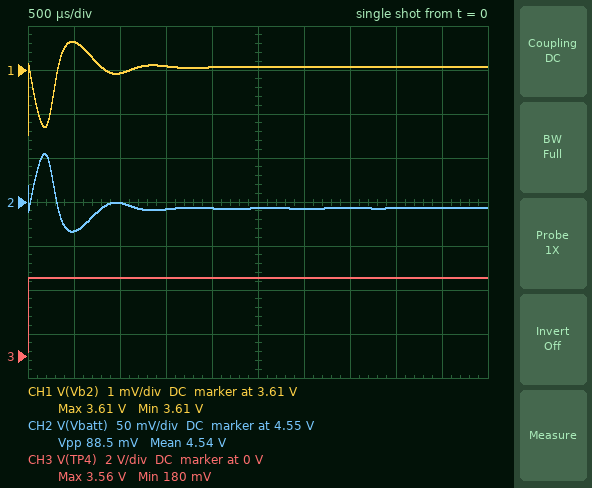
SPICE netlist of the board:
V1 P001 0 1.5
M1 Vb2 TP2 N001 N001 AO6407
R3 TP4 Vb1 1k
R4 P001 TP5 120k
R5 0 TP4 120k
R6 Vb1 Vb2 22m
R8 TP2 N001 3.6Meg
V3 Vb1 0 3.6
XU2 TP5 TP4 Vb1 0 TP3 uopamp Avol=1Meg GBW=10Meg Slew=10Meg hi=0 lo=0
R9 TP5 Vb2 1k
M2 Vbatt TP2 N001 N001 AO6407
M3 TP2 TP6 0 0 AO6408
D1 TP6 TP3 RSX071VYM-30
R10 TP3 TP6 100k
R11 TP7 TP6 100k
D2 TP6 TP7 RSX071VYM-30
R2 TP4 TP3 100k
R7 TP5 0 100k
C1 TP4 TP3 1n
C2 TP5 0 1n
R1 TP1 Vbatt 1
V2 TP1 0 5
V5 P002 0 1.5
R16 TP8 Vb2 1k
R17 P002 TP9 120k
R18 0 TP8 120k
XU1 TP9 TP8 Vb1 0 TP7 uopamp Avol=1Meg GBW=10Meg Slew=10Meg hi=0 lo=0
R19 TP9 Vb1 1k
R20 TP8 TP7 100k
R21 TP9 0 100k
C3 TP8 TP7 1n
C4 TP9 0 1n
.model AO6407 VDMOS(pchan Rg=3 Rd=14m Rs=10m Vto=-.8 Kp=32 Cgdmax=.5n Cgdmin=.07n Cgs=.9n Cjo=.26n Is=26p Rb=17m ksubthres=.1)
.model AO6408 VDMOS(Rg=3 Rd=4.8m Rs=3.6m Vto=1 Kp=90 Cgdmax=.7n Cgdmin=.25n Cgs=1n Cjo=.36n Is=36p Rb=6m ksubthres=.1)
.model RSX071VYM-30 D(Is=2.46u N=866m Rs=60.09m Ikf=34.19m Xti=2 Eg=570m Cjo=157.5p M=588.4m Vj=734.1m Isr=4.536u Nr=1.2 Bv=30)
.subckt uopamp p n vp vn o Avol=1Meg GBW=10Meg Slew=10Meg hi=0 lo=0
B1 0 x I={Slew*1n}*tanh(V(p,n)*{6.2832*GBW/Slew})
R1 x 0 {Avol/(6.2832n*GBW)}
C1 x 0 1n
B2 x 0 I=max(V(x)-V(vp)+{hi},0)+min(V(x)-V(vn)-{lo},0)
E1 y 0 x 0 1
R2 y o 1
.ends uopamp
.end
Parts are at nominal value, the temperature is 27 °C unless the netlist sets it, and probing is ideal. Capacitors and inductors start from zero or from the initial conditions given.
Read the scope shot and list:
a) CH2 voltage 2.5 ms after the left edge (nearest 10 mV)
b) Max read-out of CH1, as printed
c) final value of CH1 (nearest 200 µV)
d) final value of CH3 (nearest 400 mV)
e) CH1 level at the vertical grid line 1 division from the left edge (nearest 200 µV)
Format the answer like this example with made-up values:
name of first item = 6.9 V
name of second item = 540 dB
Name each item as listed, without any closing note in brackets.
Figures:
CH2 voltage 2.5 ms after the left edge = 4.54 V
Max read-out of CH1, as printed = 3.61 V
final value of CH1 = 3.6100 V
final value of CH3 = 3.6 V
CH1 level at the vertical grid line 1 division from the left edge = 3.6106 V
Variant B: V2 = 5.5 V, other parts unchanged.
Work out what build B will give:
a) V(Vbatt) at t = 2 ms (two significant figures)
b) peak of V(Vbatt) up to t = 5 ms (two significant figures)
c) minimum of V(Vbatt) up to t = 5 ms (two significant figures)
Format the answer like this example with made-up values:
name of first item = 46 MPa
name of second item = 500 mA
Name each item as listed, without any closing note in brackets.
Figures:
V(Vbatt) at t = 2 ms = 5.0 V
peak of V(Vbatt) up to t = 5 ms = 5.1 V
minimum of V(Vbatt) up to t = 5 ms = 4.8 V
